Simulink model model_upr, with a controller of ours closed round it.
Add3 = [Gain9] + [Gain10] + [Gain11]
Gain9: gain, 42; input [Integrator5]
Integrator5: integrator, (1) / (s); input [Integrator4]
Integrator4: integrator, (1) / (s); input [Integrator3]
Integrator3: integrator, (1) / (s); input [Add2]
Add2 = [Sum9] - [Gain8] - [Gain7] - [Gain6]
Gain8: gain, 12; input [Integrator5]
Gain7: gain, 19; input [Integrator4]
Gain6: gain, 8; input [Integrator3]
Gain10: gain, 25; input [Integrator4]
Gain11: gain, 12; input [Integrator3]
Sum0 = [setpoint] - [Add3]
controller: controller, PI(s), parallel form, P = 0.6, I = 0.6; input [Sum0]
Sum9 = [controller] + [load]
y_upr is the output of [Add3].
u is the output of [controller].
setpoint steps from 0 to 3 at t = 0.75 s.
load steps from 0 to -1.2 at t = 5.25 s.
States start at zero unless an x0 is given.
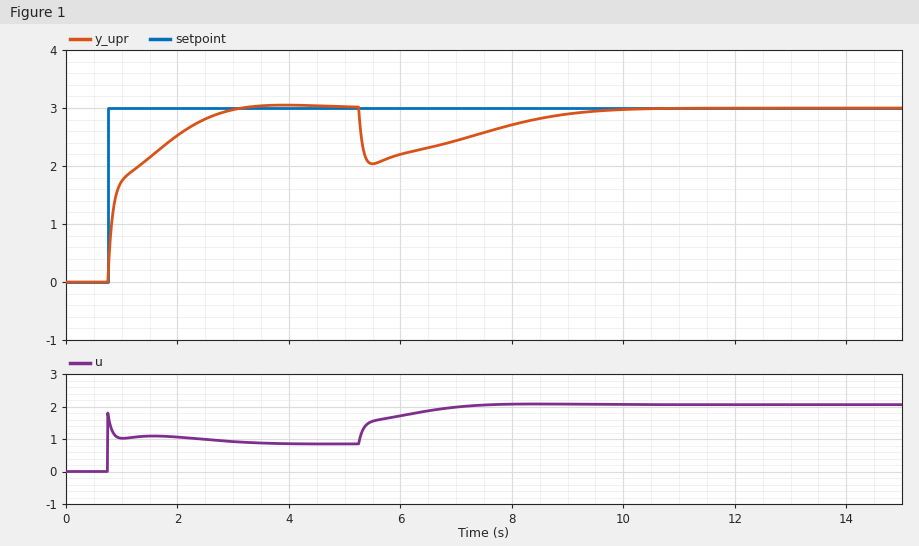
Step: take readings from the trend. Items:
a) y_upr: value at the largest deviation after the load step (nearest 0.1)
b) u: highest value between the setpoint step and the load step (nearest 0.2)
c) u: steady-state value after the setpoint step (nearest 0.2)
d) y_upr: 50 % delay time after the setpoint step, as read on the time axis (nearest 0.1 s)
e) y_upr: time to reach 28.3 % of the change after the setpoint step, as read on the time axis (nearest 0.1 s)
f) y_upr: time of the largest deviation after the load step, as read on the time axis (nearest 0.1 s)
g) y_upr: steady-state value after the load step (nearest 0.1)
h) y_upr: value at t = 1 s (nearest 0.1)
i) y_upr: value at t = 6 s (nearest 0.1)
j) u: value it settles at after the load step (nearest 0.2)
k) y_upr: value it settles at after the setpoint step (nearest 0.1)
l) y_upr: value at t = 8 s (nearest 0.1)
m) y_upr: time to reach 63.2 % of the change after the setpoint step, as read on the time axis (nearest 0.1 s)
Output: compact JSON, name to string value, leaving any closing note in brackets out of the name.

{"y_upr: value at the largest deviation after the load step": "2.0", "u: highest value between the setpoint step and the load step": "1.8", "u: steady-state value after the setpoint step": "0.8", "y_upr: 50 % delay time after the setpoint step, as read on the time axis": "0.9 s", "y_upr: time to reach 28.3 % of the change after the setpoint step, as read on the time axis": "0.8 s", "y_upr: time of the largest deviation after the load step, as read on the time axis": "5.5 s", "y_upr: steady-state value after the load step": "3.0", "y_upr: value at t = 1 s": "1.7", "y_upr: value at t = 6 s": "2.2", "u: value it settles at after the load step": "2.0", "y_upr: value it settles at after the setpoint step": "3.0", "y_upr: value at t = 8 s": "2.7", "y_upr: time to reach 63.2 % of the change after the setpoint step, as read on the time axis": "1.2 s"}
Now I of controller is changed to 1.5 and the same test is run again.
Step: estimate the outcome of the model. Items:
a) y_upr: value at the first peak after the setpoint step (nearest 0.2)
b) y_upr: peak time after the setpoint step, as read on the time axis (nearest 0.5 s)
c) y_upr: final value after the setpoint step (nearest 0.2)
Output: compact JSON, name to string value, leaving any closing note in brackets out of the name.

{"y_upr: value at the first peak after the setpoint step": "3.2", "y_upr: peak time after the setpoint step, as read on the time axis": "3.0 s", "y_upr: final value after the setpoint step": "3.0"}
